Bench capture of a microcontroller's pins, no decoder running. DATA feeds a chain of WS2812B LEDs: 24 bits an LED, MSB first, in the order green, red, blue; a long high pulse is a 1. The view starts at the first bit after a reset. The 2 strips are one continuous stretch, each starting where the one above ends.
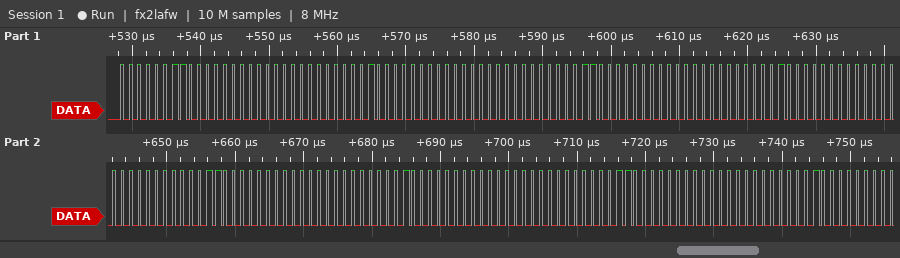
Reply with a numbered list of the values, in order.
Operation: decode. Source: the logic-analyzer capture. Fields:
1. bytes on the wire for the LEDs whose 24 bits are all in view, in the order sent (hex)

1. 03 00 00 04 00 00 03 00 00 04 00 00 03 00 00 04 00 00 03 00 00
